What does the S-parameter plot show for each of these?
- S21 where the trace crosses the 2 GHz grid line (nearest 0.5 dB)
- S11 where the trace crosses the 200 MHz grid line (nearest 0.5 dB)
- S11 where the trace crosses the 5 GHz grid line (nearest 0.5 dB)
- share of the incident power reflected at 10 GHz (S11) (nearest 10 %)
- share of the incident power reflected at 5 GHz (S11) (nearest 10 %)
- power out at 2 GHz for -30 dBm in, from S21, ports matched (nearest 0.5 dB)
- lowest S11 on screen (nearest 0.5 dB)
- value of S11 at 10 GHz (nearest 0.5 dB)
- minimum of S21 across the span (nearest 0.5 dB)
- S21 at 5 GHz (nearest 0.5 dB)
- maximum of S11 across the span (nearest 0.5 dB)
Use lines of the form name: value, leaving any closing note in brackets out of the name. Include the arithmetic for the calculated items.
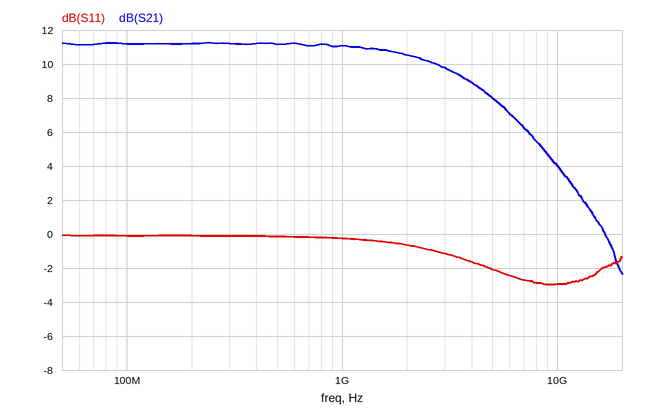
S21 where the trace crosses the 2 GHz grid line: 10.5 dB
S11 where the trace crosses the 200 MHz grid line: 0.0 dB
S11 where the trace crosses the 5 GHz grid line: -2.0 dB
share of the incident power reflected at 10 GHz (S11): 10^(-3/10) ≈ 50 %
share of the incident power reflected at 5 GHz (S11): 10^(-2/10) ≈ 63.1 %, so 60 % to the nearest 10 %
power out at 2 GHz for -30 dBm in, from S21, ports matched: -30 dBm + (10.5 dB) = -19.5 dBm
lowest S11 on screen: -3.0 dB
value of S11 at 10 GHz: -3.0 dB
minimum of S21 across the span: -2.5 dB
S21 at 5 GHz: 8.0 dB
maximum of S11 across the span: 0.0 dB
